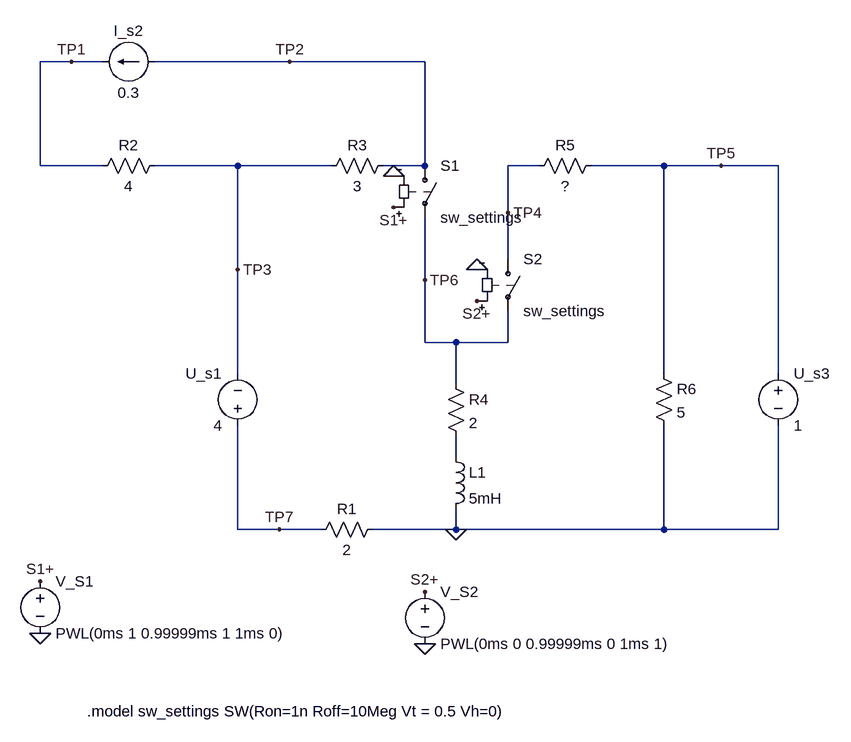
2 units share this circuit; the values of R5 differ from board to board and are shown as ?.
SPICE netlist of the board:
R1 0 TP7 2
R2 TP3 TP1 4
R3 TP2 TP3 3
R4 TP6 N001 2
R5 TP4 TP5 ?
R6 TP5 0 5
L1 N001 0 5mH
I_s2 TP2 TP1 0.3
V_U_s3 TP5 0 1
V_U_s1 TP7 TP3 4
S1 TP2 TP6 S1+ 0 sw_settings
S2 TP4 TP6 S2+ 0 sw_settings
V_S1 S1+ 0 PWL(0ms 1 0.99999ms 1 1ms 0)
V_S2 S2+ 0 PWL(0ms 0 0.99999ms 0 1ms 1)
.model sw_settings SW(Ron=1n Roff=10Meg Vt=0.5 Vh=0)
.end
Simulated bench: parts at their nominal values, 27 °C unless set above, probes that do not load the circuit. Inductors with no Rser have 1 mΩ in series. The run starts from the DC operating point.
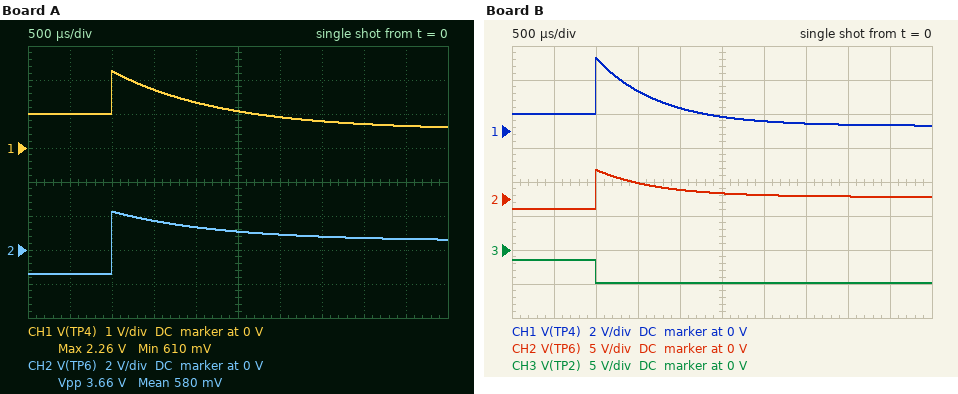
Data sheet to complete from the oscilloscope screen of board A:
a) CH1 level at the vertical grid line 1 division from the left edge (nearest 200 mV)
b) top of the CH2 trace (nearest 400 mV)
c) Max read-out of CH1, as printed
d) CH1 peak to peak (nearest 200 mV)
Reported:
1.0 V
2.4 V
2.26 V
1.6 V
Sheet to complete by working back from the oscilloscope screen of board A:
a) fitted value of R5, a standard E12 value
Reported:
1.8 Ω
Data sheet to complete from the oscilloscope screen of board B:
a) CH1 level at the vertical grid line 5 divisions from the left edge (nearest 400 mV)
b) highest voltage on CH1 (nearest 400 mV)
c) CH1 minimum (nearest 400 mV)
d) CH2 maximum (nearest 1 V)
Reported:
800 mV
4.4 V
400 mV
4 V
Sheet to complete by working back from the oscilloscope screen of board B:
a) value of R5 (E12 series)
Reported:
4.7 Ω
